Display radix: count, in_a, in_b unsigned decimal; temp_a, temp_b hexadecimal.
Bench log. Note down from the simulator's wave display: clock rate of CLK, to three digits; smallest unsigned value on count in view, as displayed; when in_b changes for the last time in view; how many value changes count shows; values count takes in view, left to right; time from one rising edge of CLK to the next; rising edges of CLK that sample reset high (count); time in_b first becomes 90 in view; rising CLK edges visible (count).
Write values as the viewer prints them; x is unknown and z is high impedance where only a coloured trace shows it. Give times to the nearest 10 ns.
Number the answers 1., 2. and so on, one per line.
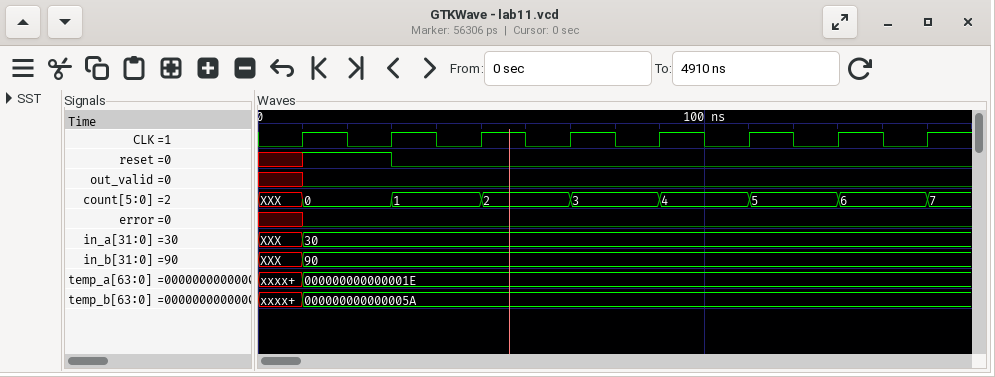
1. 50.0 MHz
2. 0
3. 10 ns
4. 8
5. XXX, 0, 1, 2, 3, 4, 5, 6, 7
6. 20 ns
7. 1
8. 10 ns
9. 8
